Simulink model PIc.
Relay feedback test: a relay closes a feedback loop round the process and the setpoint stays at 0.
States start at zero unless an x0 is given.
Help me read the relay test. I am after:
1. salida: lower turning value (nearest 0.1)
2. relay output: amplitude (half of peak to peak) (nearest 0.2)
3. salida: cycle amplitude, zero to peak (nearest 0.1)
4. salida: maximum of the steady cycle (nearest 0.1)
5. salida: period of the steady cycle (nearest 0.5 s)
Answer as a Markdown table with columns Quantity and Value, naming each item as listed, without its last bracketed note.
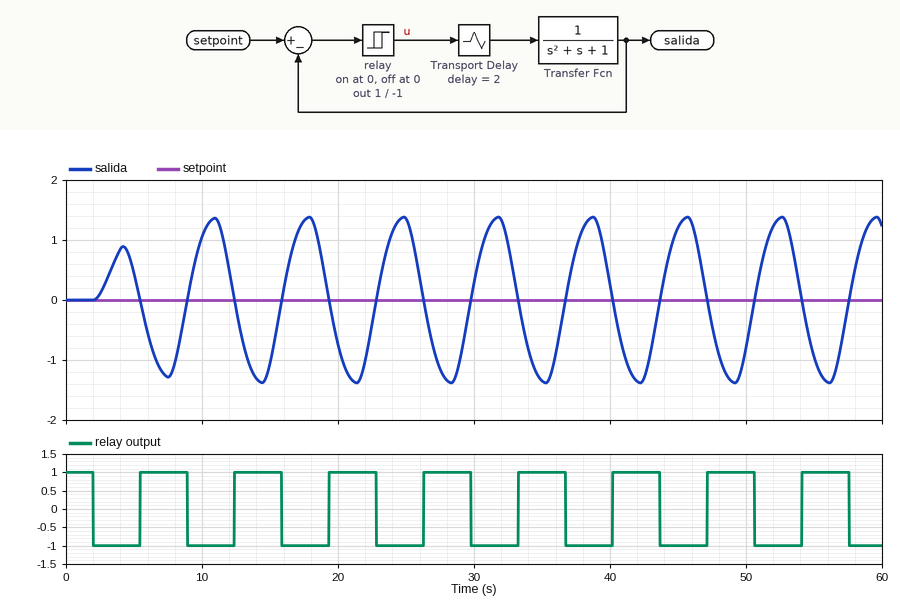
| Quantity | Value |
|---|---|
| salida: lower turning value | -1.4 |
| relay output: amplitude (half of peak to peak) | 1.0 |
| salida: cycle amplitude, zero to peak | 1.4 |
| salida: maximum of the steady cycle | 1.4 |
| salida: period of the steady cycle | 7.0 s |
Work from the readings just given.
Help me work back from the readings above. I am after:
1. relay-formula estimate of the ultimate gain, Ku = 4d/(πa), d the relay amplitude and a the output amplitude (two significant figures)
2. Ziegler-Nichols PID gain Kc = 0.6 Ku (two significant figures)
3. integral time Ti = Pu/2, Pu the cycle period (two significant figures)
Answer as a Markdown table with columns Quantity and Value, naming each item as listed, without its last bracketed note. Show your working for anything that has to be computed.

| Quantity | Value |
|---|---|
| relay-formula estimate of the ultimate gain, Ku = 4d/(πa), d the relay amplitude and a the output amplitude | 4 × 1 / (π × 1.4) = 0.91 |
| Ziegler-Nichols PID gain Kc = 0.6 Ku | 0.6 × 0.91 = 0.55 |
| integral time Ti = Pu/2, Pu the cycle period | 7 / 2 = 3.5 s |
